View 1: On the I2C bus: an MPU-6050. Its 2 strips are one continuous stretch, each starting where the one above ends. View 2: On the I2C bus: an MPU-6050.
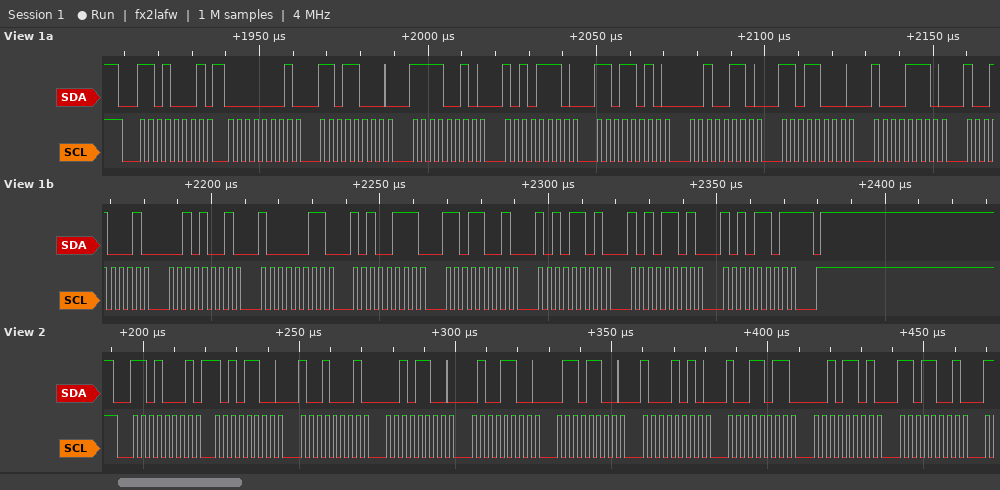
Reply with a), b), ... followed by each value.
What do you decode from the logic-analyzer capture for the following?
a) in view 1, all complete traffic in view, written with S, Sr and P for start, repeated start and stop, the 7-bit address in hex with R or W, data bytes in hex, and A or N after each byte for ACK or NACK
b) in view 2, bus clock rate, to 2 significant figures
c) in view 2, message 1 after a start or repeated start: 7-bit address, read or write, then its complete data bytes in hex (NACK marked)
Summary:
a) S 68R A 01 A D8 A F2 A AE A DA A 26 A D8 A 8E A 91 A 29 A 83 A A7 A D9 A AD A AD A AD N P
b) 400 kHz
c) 0x68 read: AC 91 2C 4C 6C 8A 9B 2D D9
